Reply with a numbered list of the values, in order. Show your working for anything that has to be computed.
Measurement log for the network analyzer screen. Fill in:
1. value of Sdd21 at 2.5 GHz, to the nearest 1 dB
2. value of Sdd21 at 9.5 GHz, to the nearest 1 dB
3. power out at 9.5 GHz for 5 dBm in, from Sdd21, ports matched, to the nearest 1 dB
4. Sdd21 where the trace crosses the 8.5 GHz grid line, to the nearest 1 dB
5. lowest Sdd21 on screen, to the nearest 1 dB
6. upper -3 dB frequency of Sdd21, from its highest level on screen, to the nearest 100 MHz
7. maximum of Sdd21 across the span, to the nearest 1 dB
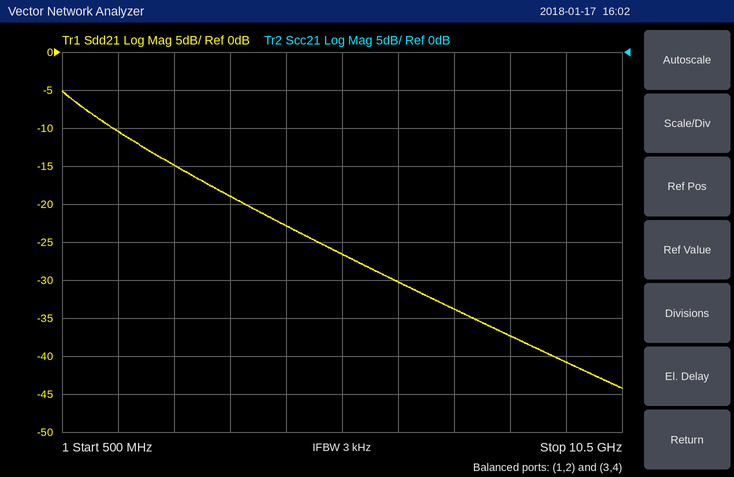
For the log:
1. -15 dB
2. -41 dB
3. 5 dBm + (-41 dB) = -36 dBm
4. -37 dB
5. -44 dB
6. 1.0 GHz
7. -5 dB
